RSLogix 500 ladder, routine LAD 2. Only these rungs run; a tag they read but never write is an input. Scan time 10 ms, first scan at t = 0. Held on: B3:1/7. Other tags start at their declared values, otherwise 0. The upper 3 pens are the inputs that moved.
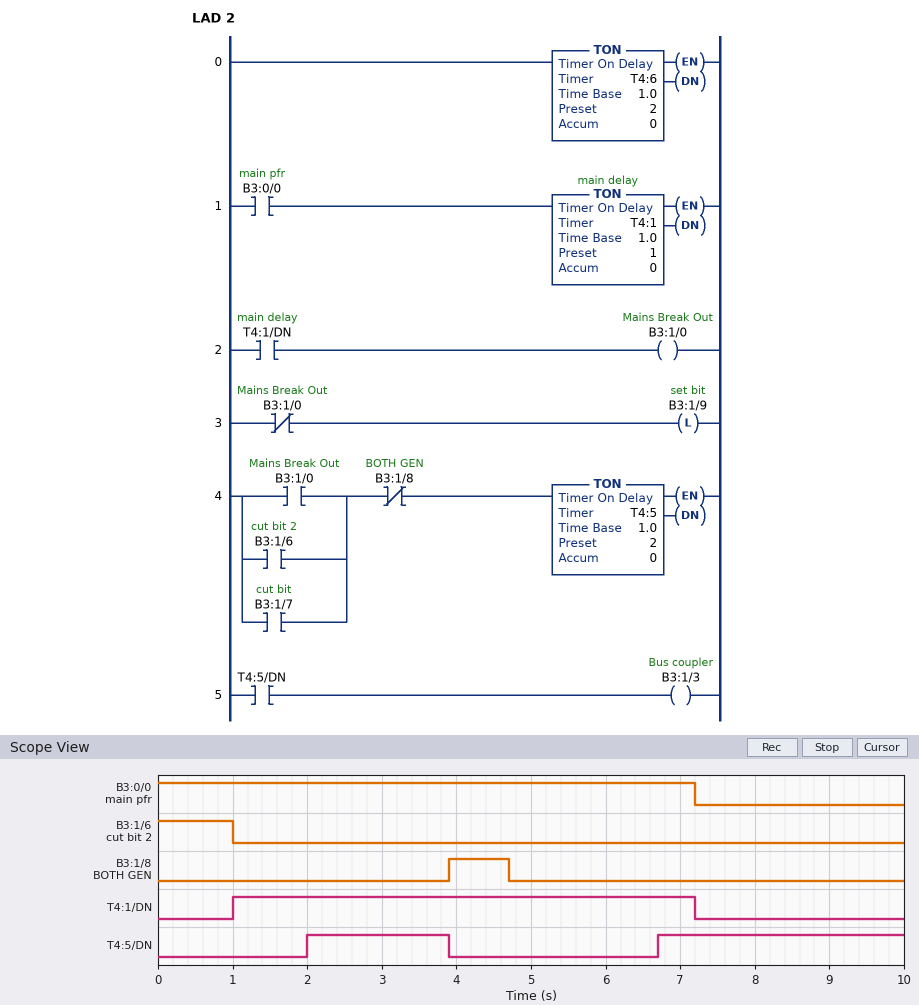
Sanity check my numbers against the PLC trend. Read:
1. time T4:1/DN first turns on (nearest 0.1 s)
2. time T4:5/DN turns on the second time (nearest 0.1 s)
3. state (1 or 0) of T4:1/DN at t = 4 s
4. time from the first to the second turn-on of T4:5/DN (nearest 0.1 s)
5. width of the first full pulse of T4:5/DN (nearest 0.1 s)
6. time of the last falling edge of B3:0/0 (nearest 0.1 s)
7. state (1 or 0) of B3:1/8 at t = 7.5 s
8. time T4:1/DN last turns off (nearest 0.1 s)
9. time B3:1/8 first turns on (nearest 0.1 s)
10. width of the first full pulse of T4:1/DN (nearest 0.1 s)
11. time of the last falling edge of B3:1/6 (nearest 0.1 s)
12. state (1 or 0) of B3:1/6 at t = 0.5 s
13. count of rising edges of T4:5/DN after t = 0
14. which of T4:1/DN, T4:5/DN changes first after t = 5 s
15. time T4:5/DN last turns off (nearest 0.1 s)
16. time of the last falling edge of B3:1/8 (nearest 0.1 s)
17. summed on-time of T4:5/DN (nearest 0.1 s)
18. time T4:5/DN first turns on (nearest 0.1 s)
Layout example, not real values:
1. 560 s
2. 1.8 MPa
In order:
1. 1.0 s
2. 6.7 s
3. 1
4. 4.7 s
5. 1.9 s
6. 7.2 s
7. 0
8. 7.2 s
9. 3.9 s
10. 6.2 s
11. 1.0 s
12. 1
13. 2
14. T4:5/DN
15. 3.9 s
16. 4.7 s
17. 5.2 s
18. 2.0 s
